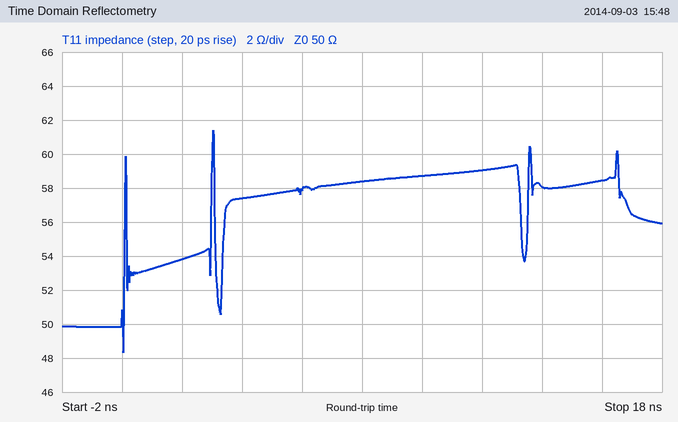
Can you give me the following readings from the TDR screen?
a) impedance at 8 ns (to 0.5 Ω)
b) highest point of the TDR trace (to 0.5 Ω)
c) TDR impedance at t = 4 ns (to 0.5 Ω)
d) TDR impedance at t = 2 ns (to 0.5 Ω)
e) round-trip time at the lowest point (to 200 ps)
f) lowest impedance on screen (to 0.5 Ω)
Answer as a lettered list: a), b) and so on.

a) 58.5 Ω
b) 61.5 Ω
c) 57.5 Ω
d) 54.0 Ω
e) 0.0 ns
f) 48.5 Ω
